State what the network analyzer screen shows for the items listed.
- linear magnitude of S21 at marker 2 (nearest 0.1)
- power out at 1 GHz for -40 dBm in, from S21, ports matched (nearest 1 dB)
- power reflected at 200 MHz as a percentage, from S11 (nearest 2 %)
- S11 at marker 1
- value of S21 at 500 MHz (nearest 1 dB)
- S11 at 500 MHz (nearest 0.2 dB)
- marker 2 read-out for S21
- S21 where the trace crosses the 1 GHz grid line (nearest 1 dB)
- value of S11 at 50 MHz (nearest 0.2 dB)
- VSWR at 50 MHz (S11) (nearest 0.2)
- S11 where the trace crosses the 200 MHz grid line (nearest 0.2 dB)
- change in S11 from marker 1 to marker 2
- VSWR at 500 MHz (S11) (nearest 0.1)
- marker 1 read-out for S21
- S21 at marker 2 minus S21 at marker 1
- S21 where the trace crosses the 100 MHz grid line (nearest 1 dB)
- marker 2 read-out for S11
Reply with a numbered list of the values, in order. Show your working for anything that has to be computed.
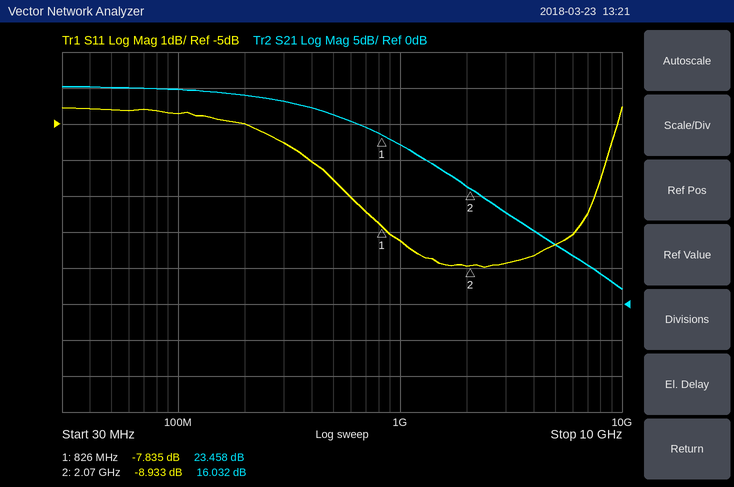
1. 10^(16.032/20) ≈ 6.3
2. -40 dBm + (22 dB) = -18 dBm
3. 10^(-5/10) ≈ 32 %
4. -7.835 dB
5. 26 dB
6. -6.6 dB
7. 16.032 dB
8. 22 dB
9. -4.6 dB
10. |Γ| = 10^(-4.6/20) = 0.5888; VSWR = (1 + 0.5888)/(1 − 0.5888) ≈ 3.86, so 3.8 to the nearest 0.2
11. -5.0 dB
12. -8.933 − (-7.835) = -1.098 dB
13. |Γ| = 10^(-6.6/20) = 0.4677; VSWR = (1 + 0.4677)/(1 − 0.4677) ≈ 2.8
14. 23.458 dB
15. 16.032 − (23.458) = -7.426 dB
16. 30 dB
17. -8.933 dB
